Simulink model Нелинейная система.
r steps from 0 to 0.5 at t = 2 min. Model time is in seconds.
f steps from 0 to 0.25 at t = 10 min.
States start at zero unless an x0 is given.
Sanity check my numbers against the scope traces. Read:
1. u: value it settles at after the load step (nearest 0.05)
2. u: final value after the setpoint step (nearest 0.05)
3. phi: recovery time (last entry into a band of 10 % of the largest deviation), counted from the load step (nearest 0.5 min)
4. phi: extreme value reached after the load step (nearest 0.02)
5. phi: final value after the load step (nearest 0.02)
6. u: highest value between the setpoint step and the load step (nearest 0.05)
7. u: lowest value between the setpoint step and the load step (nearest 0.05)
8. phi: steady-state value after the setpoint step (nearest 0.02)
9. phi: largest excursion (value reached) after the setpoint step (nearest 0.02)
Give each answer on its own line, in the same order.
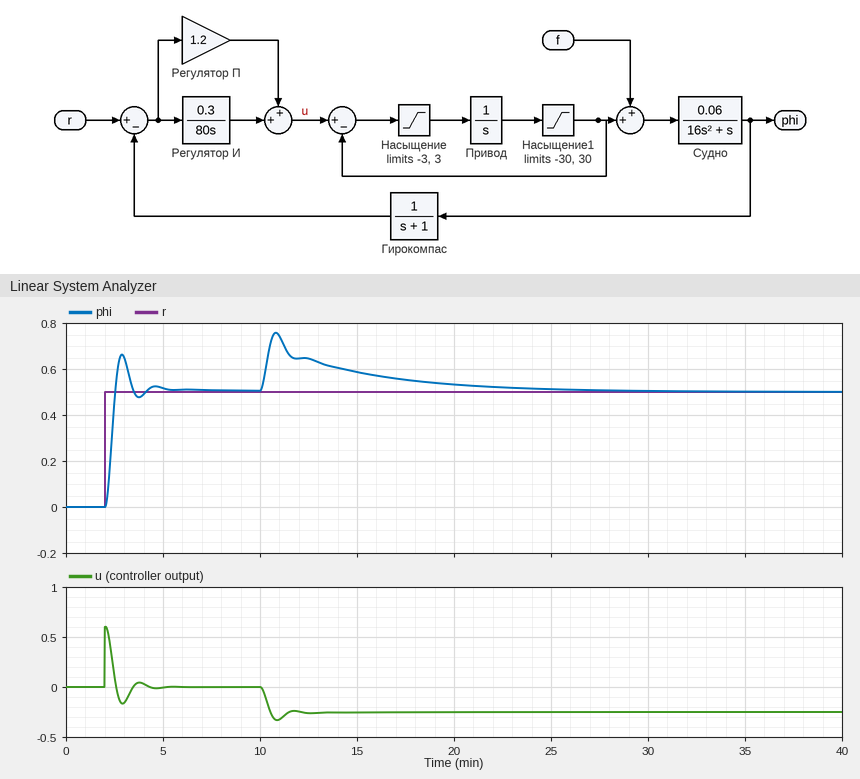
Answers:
-0.25
0.00
11.5 min
0.76
0.50
0.60
-0.15
0.50
0.66
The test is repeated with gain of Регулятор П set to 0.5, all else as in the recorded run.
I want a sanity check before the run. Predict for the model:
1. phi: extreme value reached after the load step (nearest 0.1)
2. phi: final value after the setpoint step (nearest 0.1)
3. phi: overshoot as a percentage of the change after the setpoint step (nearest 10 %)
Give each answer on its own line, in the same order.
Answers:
1.0
0.5
30 %
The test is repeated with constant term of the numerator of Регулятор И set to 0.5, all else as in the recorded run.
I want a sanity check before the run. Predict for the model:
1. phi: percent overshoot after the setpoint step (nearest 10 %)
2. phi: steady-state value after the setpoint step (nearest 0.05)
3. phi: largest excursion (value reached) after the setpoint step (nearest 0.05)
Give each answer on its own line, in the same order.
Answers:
40 %
0.50
0.70
